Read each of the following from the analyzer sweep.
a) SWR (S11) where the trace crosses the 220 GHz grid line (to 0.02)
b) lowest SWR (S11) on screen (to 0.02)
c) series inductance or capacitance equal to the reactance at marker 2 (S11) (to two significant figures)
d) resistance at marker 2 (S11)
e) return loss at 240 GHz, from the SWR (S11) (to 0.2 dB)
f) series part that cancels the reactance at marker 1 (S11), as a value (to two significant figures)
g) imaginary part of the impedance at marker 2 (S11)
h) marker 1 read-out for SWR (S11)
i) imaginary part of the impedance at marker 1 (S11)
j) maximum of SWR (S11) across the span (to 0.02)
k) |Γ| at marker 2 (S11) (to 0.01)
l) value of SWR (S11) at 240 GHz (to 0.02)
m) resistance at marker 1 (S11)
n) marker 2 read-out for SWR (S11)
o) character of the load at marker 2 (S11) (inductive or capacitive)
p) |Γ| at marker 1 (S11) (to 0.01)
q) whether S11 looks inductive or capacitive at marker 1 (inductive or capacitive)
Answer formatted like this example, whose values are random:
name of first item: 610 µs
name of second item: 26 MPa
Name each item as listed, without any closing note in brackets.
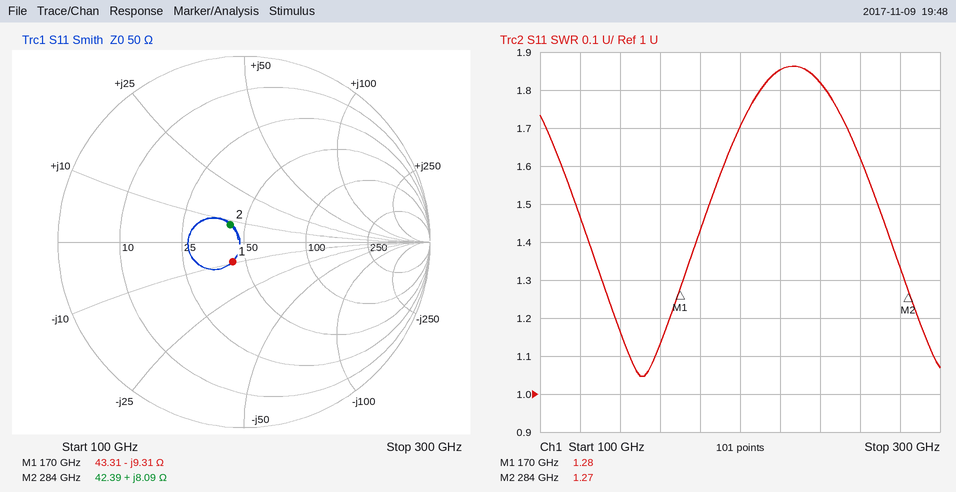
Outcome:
SWR (S11) where the trace crosses the 220 GHz grid line: 1.86
lowest SWR (S11) on screen: 1.04
series inductance or capacitance equal to the reactance at marker 2 (S11): 4.5 pH
resistance at marker 2: 42.39 Ω
return loss at 240 GHz, from the SWR (S11): 10.8 dB
series part that cancels the reactance at marker 1 (S11), as a value: 8.7 pH
imaginary part of the impedance at marker 2: +8.09 Ω
marker 1 read-out for SWR: 1.28
imaginary part of the impedance at marker 1: -9.31 Ω
maximum of SWR (S11) across the span: 1.86
|Γ| at marker 2 (S11): 0.12
value of SWR (S11) at 240 GHz: 1.82
resistance at marker 1: 43.31 Ω
marker 2 read-out for SWR: 1.27
character of the load at marker 2 (S11): inductive
|Γ| at marker 1 (S11): 0.12
whether S11 looks inductive or capacitive at marker 1: capacitive
